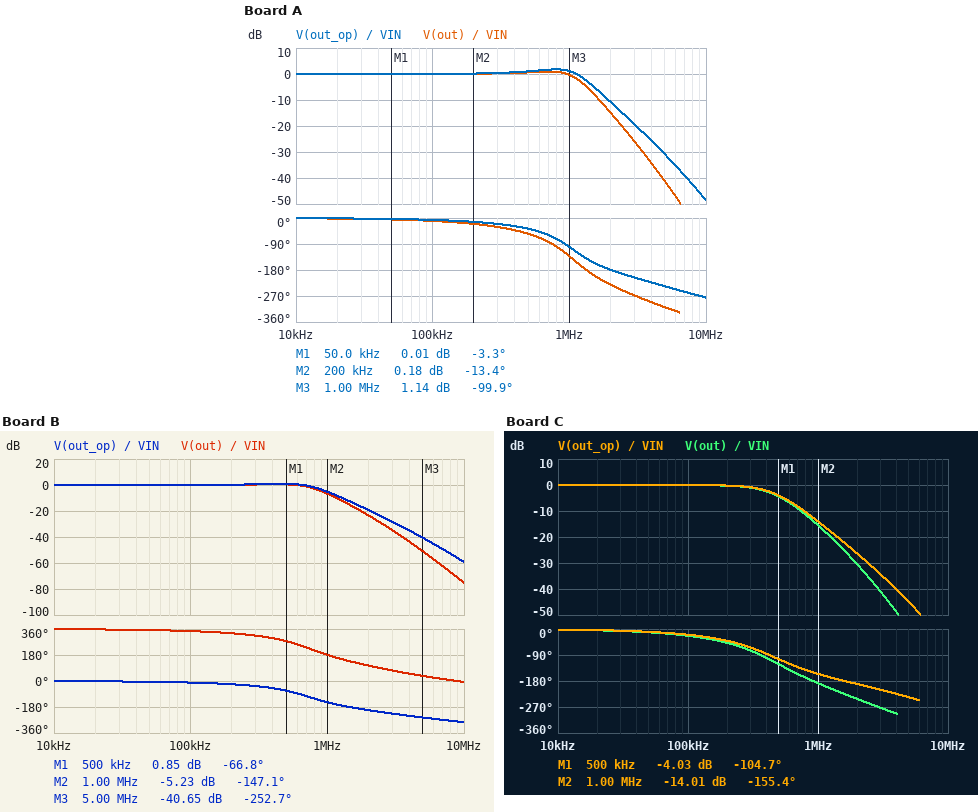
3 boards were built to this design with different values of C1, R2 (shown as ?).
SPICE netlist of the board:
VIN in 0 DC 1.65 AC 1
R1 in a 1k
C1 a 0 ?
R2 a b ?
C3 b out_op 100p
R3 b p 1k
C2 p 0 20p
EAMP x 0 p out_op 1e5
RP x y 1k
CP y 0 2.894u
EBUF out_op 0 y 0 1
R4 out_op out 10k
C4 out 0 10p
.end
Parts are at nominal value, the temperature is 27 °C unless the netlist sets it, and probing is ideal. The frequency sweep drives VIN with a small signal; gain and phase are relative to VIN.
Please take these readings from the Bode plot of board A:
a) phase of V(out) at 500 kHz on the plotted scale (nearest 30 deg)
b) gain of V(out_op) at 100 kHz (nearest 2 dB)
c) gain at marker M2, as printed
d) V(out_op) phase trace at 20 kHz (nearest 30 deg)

-60 deg
0 dB
0.18 dB
0 deg
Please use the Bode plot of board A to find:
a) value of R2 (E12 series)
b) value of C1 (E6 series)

3.3 kΩ
47 pF
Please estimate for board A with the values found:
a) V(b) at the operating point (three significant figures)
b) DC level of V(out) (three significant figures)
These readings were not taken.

1.65 V
1.65 V
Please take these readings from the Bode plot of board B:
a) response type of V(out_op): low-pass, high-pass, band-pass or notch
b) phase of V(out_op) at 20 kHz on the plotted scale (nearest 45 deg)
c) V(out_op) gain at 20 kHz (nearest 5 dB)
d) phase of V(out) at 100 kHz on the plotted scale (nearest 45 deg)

low-pass
0 deg
0 dB
360 deg
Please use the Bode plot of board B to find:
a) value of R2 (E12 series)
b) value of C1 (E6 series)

8.2 kΩ
68 pF
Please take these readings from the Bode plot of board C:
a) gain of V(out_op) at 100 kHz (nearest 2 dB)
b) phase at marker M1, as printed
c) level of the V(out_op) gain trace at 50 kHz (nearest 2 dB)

0 dB
-104.7 deg
0 dB
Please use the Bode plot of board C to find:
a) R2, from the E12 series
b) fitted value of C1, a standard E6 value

22 kΩ
33 pF
